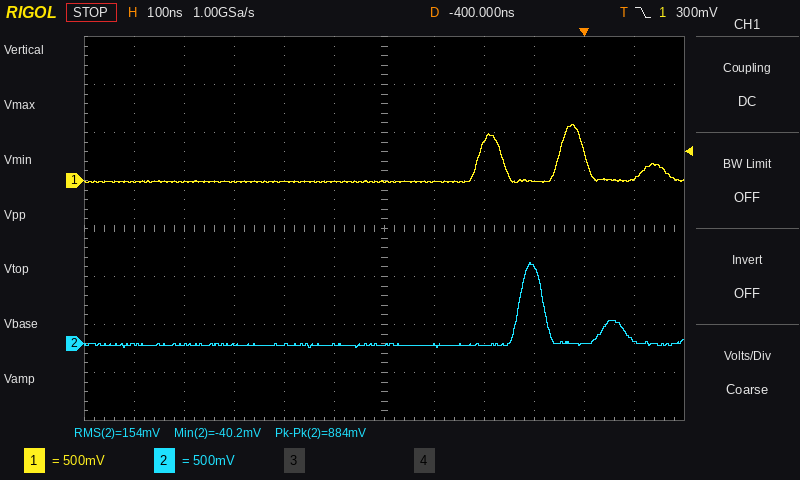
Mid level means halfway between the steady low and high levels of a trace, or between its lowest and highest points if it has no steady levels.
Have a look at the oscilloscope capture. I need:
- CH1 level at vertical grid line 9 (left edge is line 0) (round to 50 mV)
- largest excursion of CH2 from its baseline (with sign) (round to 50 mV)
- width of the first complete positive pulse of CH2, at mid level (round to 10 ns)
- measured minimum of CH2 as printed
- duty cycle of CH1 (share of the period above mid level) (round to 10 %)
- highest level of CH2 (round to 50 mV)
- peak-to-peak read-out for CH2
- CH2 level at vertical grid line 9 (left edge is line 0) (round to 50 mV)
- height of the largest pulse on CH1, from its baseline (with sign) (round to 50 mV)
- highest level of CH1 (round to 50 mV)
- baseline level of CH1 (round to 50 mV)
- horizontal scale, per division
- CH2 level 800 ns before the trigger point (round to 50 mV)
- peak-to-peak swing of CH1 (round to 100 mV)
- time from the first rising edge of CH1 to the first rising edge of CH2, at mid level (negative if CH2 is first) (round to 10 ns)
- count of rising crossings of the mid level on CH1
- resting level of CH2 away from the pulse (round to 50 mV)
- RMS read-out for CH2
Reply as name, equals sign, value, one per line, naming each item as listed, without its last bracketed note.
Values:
CH1 level at vertical grid line 9 (left edge is line 0) = 0 mV
largest excursion of CH2 from its baseline (with sign) = +850 mV
width of the first complete positive pulse of CH2, at mid level = 50 ns
measured minimum of CH2 as printed = -40.2 mV
duty cycle of CH1 (share of the period above mid level) = 30 %
highest level of CH2 = 850 mV
peak-to-peak read-out for CH2 = 884 mV
CH2 level at vertical grid line 9 (left edge is line 0) = 800 mV
height of the largest pulse on CH1, from its baseline (with sign) = +600 mV
highest level of CH1 = 600 mV
baseline level of CH1 = 0 mV
horizontal scale, per division = 100 ns
CH2 level 800 ns before the trigger point = 0 mV
peak-to-peak swing of CH1 = 600 mV
time from the first rising edge of CH1 to the first rising edge of CH2, at mid level (negative if CH2 is first) = +80 ns
count of rising crossings of the mid level on CH1 = 2
resting level of CH2 away from the pulse = 0 mV
RMS read-out for CH2 = 154 mV
